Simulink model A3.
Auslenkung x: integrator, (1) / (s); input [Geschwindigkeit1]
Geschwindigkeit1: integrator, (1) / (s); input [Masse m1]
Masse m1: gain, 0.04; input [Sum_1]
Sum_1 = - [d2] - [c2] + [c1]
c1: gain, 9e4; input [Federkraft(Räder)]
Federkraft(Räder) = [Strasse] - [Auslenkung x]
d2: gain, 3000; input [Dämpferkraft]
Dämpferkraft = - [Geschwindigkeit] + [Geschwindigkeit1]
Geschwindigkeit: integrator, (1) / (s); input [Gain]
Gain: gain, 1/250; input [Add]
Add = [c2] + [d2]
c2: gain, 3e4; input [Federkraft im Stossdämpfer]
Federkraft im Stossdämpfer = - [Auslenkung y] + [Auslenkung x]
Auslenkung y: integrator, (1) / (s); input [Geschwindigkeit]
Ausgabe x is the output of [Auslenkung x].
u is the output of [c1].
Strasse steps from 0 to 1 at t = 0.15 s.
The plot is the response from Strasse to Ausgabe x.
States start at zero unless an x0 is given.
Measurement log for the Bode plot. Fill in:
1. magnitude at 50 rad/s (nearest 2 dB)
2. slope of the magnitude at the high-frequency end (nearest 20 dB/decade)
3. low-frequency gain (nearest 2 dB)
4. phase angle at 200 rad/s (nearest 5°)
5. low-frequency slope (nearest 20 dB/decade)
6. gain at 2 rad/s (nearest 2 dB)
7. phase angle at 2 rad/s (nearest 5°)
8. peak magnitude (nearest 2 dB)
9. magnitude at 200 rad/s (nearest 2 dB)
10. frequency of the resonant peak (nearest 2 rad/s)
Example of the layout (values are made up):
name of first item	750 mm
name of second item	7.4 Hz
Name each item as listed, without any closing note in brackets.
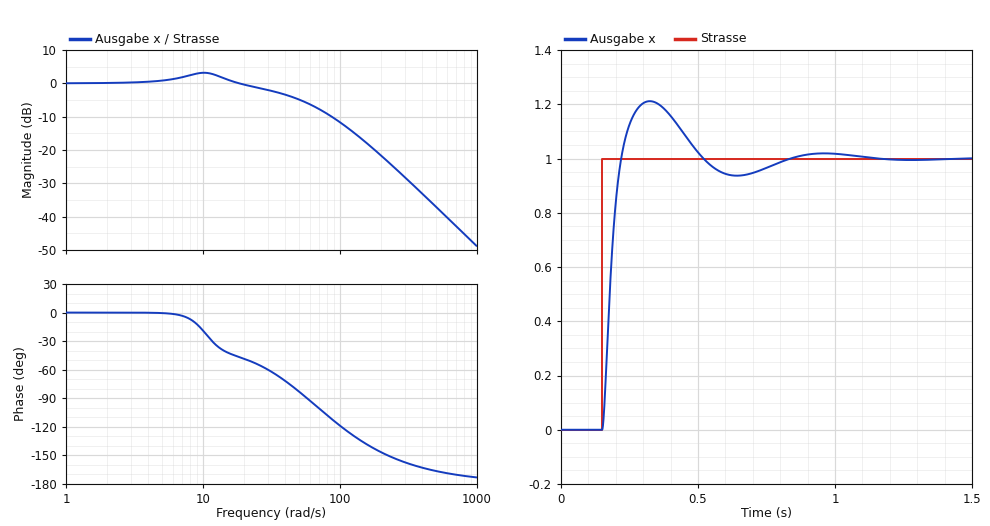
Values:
magnitude at 50 rad/s	-4 dB
slope of the magnitude at the high-frequency end	-40 dB/decade
low-frequency gain	0 dB
phase angle at 200 rad/s	-145°
low-frequency slope	0 dB/decade
gain at 2 rad/s	0 dB
phase angle at 2 rad/s	0°
peak magnitude	4 dB
magnitude at 200 rad/s	-22 dB
frequency of the resonant peak	10 rad/s
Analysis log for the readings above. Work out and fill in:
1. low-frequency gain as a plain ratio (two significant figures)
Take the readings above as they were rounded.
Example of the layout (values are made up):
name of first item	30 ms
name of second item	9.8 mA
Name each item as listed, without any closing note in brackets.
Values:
low-frequency gain as a plain ratio	1.0
